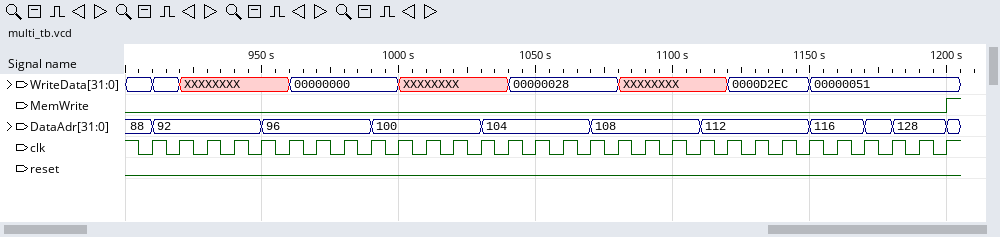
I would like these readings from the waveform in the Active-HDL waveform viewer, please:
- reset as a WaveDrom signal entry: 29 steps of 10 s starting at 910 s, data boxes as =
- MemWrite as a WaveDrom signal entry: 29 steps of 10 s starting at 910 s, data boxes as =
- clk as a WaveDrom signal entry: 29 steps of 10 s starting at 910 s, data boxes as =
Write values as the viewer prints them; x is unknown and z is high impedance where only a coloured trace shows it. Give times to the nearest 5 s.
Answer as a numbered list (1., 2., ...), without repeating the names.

1. {name: 'reset', wave: '0............................'}
2. {name: 'MemWrite', wave: '0............................'}
3. {name: 'clk', wave: 'p............................'}
